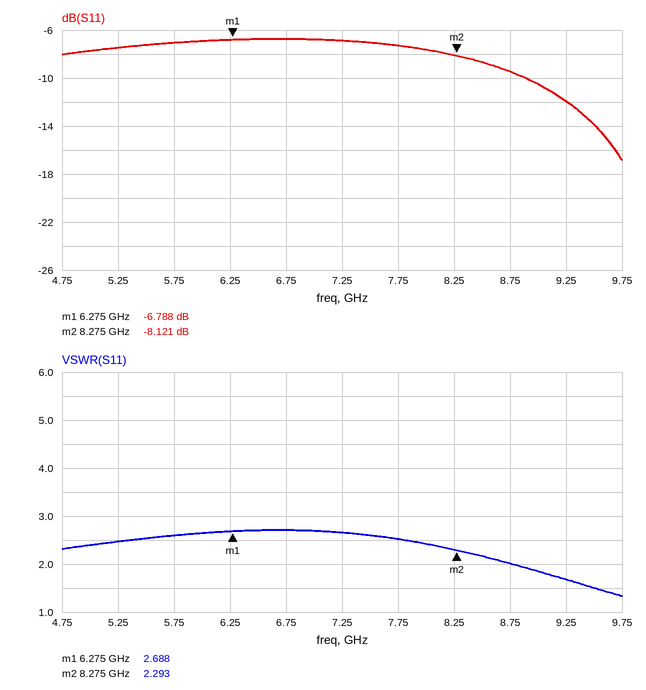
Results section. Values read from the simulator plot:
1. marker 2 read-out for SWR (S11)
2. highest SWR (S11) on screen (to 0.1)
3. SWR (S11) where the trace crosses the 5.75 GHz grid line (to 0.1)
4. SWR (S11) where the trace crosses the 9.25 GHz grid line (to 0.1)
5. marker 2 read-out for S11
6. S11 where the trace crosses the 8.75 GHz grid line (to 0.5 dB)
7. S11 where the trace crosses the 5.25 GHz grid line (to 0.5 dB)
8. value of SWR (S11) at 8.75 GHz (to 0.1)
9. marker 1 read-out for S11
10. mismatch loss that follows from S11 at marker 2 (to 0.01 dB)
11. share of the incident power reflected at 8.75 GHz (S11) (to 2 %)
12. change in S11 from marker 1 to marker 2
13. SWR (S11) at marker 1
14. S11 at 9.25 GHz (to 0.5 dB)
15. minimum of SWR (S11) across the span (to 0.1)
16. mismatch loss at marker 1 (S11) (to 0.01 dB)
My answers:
2.293
2.7
2.6
1.7
-8.121 dB
-9.5 dB
-7.5 dB
2.0
-6.788 dB
0.73 dB
12 %
-1.333 dB
2.688
-12.0 dB
1.3
1.02 dB
